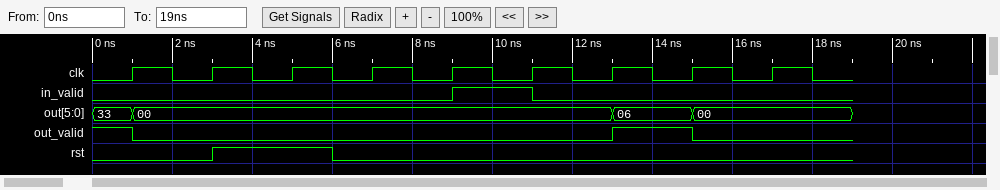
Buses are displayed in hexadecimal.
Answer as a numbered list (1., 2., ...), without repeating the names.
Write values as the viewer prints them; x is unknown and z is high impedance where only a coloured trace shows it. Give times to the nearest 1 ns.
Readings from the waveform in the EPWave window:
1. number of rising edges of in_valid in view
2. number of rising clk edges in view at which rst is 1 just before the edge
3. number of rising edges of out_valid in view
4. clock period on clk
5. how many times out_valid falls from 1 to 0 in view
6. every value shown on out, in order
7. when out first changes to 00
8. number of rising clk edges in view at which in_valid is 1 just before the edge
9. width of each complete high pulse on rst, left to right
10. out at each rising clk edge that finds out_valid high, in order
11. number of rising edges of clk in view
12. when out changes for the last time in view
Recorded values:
1. 1
2. 1
3. 1
4. 2 ns
5. 2
6. 33, 00, 06, 00
7. 1 ns
8. 1
9. 3 ns
10. 33, 06
11. 9
12. 15 ns
